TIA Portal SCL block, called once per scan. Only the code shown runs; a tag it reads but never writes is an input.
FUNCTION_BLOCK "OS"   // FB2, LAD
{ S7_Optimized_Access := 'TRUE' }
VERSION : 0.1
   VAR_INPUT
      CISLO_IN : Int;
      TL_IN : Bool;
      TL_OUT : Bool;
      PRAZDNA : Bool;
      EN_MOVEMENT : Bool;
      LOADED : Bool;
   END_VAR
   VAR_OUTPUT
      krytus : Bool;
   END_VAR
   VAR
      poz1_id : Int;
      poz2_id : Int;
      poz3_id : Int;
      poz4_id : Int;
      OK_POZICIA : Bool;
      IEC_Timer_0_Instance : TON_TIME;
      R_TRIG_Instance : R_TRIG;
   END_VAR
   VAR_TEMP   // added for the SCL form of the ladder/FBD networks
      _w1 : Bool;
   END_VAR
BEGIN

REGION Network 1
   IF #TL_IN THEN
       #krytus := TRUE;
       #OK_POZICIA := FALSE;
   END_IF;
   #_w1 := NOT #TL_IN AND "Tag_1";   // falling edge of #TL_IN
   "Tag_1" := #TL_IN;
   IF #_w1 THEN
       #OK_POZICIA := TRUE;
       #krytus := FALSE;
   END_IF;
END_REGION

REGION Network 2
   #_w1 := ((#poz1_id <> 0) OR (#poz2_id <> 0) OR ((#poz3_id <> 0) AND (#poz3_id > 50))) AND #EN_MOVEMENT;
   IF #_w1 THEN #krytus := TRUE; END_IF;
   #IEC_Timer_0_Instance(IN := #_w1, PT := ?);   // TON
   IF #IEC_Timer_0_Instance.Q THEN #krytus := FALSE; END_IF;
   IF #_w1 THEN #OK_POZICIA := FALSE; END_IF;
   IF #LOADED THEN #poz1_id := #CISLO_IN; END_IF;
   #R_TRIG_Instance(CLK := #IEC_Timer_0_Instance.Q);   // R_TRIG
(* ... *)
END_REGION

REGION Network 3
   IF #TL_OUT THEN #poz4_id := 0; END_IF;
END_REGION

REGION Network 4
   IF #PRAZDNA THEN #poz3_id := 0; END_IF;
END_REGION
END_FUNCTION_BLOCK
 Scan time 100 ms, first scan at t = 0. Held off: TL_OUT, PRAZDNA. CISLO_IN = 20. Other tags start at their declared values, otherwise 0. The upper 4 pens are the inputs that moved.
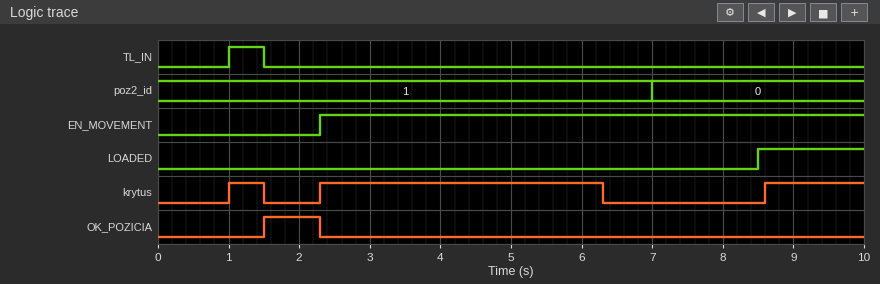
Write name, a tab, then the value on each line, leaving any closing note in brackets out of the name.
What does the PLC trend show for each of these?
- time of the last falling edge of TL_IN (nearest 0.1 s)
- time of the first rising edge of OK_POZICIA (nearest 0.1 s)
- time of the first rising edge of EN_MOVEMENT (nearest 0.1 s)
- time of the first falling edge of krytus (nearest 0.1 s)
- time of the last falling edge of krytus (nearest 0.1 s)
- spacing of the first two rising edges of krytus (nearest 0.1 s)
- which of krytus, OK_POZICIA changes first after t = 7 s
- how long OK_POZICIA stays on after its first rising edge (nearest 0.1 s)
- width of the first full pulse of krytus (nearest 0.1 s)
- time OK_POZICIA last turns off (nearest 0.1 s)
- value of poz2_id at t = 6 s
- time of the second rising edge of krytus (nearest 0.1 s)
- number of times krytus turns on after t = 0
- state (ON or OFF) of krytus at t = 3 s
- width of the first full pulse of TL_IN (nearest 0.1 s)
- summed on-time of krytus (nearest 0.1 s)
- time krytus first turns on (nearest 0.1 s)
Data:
time of the last falling edge of TL_IN	1.5 s
time of the first rising edge of OK_POZICIA	1.5 s
time of the first rising edge of EN_MOVEMENT	2.3 s
time of the first falling edge of krytus	1.5 s
time of the last falling edge of krytus	6.3 s
spacing of the first two rising edges of krytus	1.3 s
which of krytus, OK_POZICIA changes first after t = 7 s	krytus
how long OK_POZICIA stays on after its first rising edge	0.8 s
width of the first full pulse of krytus	0.5 s
time OK_POZICIA last turns off	2.3 s
value of poz2_id at t = 6 s	1
time of the second rising edge of krytus	2.3 s
number of times krytus turns on after t = 0	3
state (ON or OFF) of krytus at t = 3 s	ON
width of the first full pulse of TL_IN	0.5 s
summed on-time of krytus	5.9 s
time krytus first turns on	1.0 s
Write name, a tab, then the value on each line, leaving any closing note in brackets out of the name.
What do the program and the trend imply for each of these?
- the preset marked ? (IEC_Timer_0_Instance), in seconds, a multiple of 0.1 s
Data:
the preset marked ? (IEC_Timer_0_Instance), in seconds, a multiple of 0.1 s	4.0 s
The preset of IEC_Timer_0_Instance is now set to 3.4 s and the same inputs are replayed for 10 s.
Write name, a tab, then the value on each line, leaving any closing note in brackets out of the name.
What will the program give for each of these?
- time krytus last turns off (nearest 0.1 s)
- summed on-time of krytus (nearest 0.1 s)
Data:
time krytus last turns off	5.7 s
summed on-time of krytus	5.3 s
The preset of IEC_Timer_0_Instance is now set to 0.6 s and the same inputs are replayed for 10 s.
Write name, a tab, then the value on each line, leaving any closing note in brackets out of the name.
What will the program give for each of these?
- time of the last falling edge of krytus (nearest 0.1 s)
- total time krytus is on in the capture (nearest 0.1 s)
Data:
time of the last falling edge of krytus	9.2 s
total time krytus is on in the capture	1.7 s
